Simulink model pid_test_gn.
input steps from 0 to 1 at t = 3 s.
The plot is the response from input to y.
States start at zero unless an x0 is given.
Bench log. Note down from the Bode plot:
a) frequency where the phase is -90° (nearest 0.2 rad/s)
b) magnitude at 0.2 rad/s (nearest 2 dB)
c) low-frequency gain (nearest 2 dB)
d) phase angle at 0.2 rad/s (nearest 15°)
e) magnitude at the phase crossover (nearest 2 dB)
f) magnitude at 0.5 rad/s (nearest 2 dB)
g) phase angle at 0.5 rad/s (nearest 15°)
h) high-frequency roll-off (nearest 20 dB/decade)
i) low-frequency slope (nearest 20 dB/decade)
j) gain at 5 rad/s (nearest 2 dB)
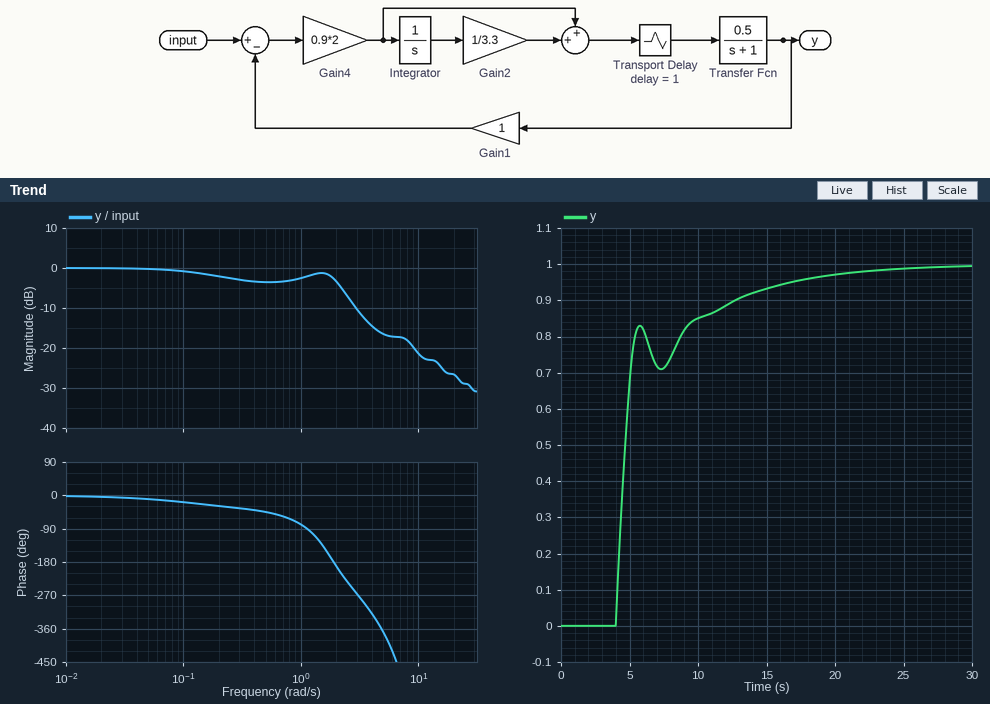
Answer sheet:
1.2 rad/s
-2 dB
0 dB
-30°
-2 dB
-4 dB
-45°
-20 dB/decade
0 dB/decade
-16 dB
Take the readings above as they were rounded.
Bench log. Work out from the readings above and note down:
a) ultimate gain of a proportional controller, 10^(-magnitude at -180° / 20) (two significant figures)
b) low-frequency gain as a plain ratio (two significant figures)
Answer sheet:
1.3
1.0
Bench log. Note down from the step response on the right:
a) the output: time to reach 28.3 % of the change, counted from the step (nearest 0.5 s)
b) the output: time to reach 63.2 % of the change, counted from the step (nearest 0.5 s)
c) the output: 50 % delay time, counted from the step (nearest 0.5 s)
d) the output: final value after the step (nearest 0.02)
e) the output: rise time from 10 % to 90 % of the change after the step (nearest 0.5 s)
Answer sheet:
1.5 s
2.0 s
1.5 s
1.00
8.5 s
